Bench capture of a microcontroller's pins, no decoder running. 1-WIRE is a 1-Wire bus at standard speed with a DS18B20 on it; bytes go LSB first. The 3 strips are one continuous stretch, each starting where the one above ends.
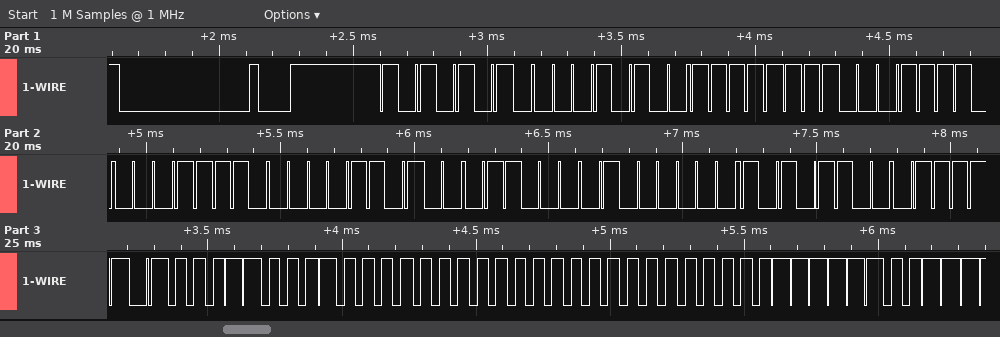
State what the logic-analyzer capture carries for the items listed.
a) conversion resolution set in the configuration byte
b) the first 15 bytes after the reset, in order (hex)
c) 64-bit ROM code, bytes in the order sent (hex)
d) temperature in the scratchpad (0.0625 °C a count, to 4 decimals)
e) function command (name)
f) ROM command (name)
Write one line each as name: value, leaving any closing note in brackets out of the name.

conversion resolution set in the configuration byte: 10 bits
the first 15 bytes after the reset, in order: 55 28 FF 78 78 B0 18 02 35 BE 18 01 00 00 3F
64-bit ROM code, bytes in the order sent: 28 FF 78 78 B0 18 02 35
temperature in the scratchpad: 17.5000 °C
function command: Read Scratchpad
ROM command: Match ROM
